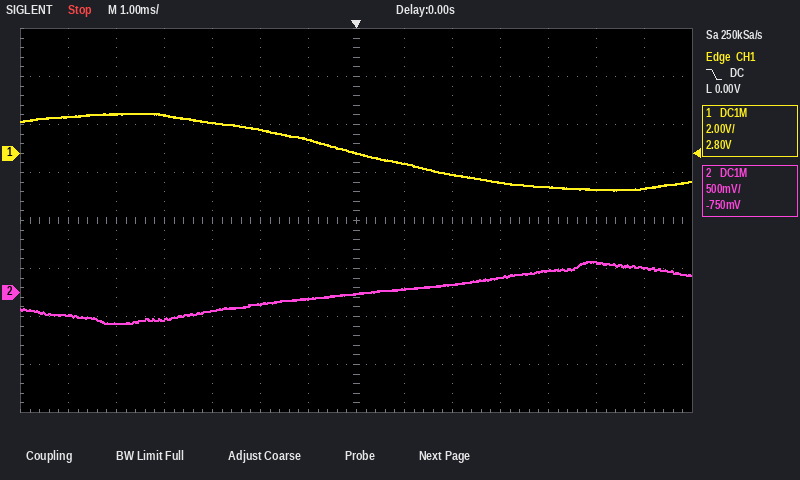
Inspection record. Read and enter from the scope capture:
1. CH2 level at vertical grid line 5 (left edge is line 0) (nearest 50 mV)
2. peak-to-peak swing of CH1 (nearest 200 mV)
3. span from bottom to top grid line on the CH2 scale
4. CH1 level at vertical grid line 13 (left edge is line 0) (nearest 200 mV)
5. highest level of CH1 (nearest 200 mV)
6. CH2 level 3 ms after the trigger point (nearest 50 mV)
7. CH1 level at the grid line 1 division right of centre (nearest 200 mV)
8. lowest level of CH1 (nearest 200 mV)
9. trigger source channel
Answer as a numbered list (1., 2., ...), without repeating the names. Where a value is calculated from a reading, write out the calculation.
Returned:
1. -100 mV
2. 1.6 V − (-1.6 V) = 3.2 V
3. 4 V
4. -1.4 V
5. 1.6 V
6. 150 mV
7. -400 mV
8. -1.6 V
9. CH1
